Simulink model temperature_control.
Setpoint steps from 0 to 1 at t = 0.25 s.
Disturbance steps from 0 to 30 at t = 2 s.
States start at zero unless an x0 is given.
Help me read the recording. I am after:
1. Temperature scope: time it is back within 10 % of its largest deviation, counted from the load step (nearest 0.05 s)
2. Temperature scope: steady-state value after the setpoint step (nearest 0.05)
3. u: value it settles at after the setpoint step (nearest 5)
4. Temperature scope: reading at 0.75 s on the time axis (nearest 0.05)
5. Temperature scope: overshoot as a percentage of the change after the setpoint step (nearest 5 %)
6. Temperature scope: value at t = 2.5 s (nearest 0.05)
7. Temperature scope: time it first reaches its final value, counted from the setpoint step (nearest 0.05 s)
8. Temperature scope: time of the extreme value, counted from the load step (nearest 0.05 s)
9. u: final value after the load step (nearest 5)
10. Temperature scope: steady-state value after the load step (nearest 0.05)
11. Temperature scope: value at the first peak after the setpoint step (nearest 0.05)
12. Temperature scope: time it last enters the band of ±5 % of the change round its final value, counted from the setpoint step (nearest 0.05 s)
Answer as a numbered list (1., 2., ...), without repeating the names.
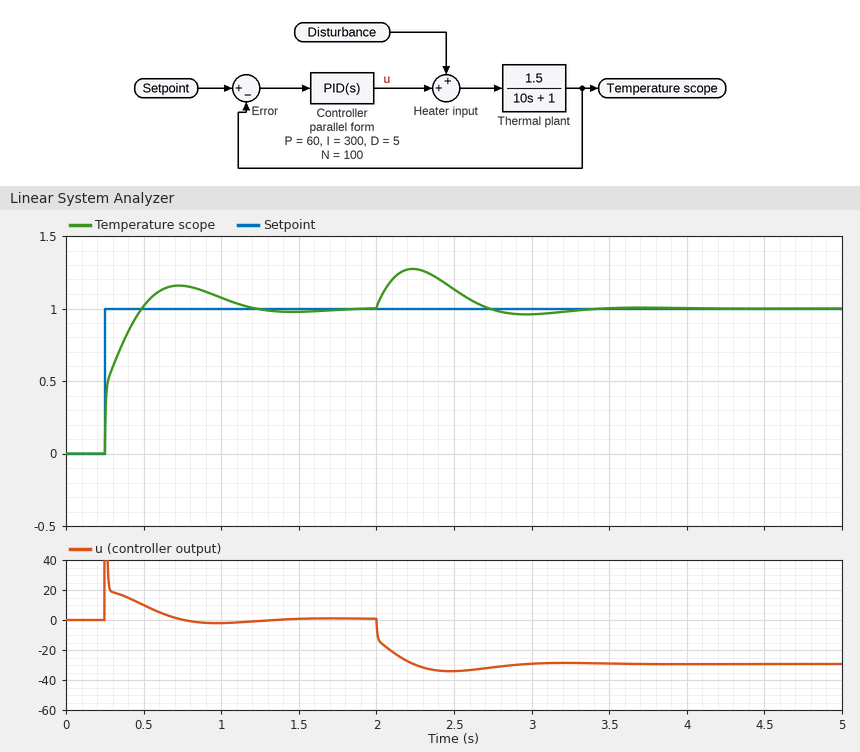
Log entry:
1. 1.15 s
2. 1.00
3. 0
4. 1.15
5. 15 %
6. 1.15
7. 0.25 s
8. 0.25 s
9. -30
10. 1.00
11. 1.15
12. 0.80 s
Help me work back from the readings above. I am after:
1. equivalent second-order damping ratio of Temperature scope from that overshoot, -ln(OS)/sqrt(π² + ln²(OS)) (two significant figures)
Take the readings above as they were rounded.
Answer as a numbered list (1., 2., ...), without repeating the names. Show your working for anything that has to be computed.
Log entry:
1. ln(0.15) = -1.897; 1.897 / sqrt(9.870 + 3.599) = 0.52
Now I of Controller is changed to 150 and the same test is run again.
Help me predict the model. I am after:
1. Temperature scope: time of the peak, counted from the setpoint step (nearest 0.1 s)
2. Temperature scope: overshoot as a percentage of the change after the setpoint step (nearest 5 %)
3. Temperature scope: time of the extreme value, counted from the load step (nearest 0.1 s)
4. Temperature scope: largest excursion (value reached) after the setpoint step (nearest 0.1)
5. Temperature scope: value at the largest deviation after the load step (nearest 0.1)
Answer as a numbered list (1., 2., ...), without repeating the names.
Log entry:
1. 0.6 s
2. 10 %
3. 0.3 s
4. 1.1
5. 1.3
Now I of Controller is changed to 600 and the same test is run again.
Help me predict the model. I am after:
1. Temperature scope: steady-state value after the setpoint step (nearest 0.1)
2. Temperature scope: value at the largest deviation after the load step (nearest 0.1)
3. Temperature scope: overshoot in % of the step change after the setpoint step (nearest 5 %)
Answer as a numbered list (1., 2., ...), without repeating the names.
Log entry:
1. 1.0
2. 1.2
3. 20 %
